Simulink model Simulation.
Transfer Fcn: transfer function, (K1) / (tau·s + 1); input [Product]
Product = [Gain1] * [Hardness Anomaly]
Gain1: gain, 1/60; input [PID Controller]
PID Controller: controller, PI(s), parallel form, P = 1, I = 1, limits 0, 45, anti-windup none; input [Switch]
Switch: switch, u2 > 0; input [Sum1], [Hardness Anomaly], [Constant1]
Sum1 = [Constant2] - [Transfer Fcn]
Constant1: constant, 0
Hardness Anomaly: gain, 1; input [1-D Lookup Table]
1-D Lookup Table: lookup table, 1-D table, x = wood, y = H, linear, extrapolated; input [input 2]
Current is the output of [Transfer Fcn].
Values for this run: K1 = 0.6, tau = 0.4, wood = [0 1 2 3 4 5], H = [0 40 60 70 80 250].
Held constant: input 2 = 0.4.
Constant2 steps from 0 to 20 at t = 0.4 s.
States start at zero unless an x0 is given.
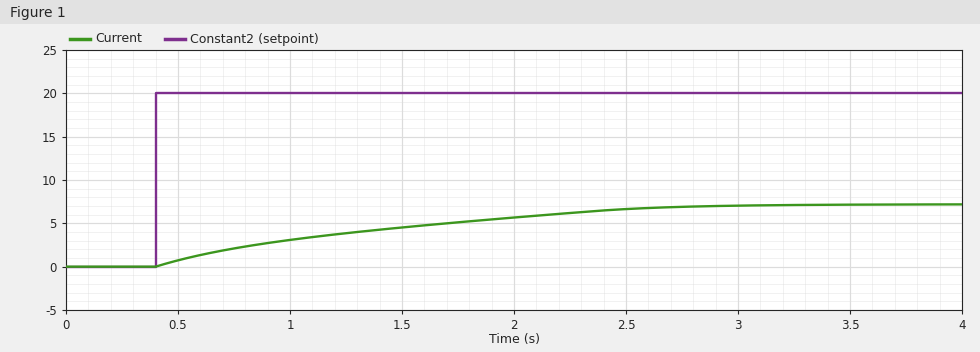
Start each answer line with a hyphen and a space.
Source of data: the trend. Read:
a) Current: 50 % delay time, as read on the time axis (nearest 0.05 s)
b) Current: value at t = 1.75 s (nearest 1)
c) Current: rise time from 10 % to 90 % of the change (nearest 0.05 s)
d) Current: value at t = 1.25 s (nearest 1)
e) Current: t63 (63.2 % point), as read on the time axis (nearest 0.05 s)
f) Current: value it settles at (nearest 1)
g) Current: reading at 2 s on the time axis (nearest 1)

- 1.15 s
- 5
- 1.90 s
- 4
- 1.50 s
- 7
- 6
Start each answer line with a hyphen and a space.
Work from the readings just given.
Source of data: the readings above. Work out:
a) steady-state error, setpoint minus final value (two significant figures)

- 13
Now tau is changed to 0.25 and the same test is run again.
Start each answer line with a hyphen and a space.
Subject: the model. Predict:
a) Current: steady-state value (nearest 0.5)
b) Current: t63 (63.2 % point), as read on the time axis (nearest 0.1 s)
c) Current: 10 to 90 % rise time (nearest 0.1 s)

- 7.0
- 1.4 s
- 1.8 s
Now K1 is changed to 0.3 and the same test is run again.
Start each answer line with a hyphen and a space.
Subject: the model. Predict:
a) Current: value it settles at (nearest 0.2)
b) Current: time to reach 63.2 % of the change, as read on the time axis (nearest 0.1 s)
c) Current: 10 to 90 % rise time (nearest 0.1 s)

- 3.6
- 1.4 s
- 1.6 s
